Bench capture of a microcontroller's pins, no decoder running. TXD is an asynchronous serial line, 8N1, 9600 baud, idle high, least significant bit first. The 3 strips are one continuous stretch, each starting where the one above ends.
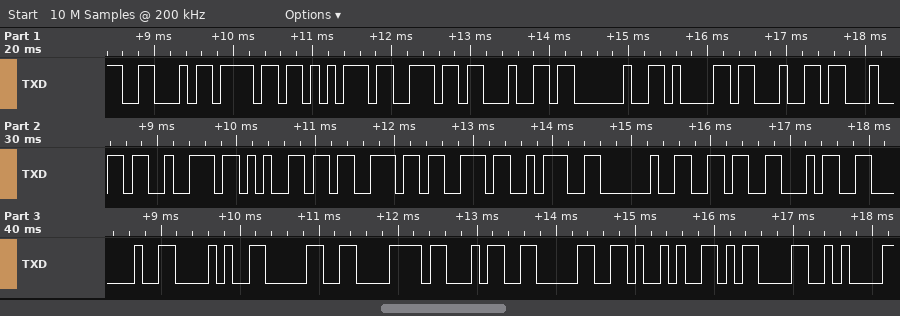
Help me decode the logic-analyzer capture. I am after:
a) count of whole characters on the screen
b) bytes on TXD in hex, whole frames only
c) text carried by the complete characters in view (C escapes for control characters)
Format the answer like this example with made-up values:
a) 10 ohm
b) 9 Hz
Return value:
a) 26
b) 0x46 0x6F 0x75 0x6E 0x64 0x20 0x61 0x64 0x64 0x72 0x65 0x73 0x73 0x3A 0x20 0x36 0x34 0x20 0x28 0x30 0x78 0x34 0x30 0x29 0x0D 0x0A
c) "Found address: 64 (0x40)\r\n"
